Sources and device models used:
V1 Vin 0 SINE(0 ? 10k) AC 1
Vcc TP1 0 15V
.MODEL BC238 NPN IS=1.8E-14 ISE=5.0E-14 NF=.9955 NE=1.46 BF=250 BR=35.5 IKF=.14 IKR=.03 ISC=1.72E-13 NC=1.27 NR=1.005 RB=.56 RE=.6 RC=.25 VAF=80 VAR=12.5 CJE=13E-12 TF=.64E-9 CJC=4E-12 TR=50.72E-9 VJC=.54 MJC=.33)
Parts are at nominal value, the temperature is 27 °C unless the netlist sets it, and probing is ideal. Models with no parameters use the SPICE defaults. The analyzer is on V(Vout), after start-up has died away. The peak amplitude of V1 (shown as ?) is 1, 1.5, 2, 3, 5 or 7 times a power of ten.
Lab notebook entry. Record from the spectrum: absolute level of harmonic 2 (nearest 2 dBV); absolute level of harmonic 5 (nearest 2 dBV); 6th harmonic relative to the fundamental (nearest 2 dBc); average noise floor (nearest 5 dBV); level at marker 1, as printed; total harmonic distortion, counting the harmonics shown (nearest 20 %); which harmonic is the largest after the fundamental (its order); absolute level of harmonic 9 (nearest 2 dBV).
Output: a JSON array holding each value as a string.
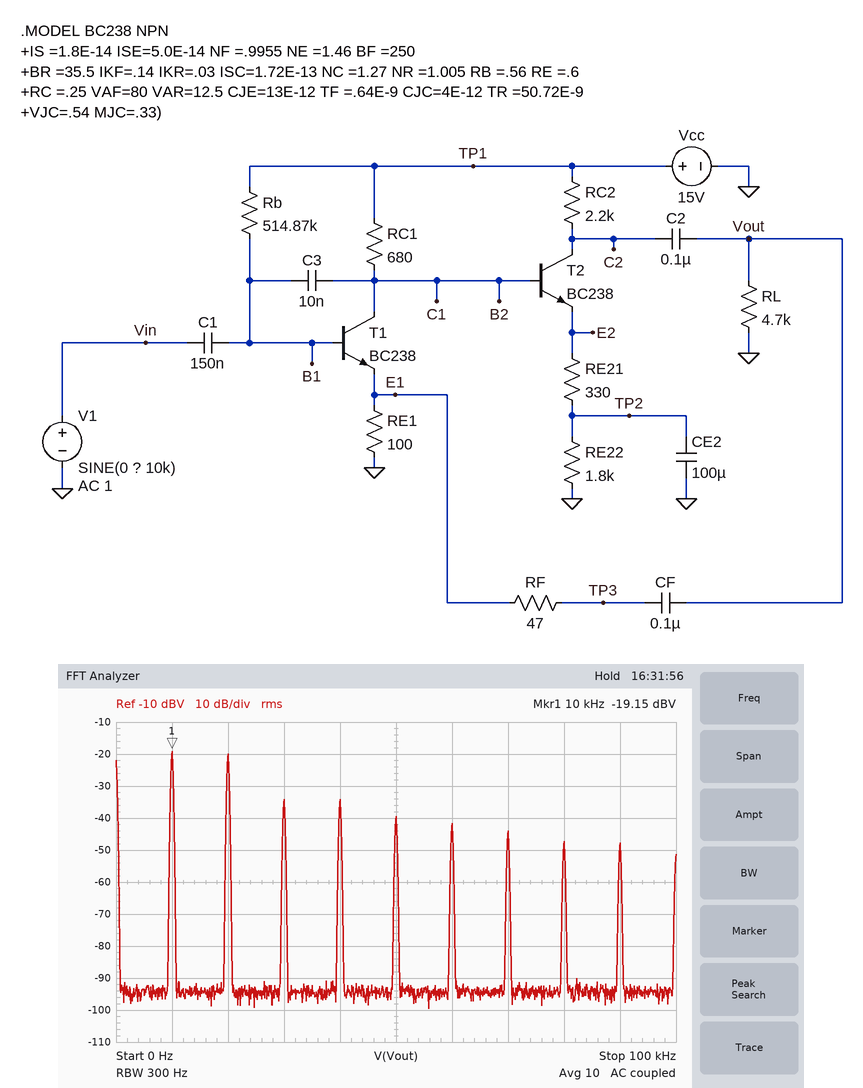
["-20 dBV", "-40 dBV", "-22 dBc", "-95 dBV", "-19.15 dBV", "100 %", "2", "-48 dBV"]
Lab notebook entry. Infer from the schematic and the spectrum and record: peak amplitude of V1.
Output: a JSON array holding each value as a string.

["500 mV"]
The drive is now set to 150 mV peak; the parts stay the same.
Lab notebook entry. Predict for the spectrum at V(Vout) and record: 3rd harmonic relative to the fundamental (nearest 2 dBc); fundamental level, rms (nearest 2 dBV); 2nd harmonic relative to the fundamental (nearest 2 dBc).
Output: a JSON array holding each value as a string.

["-34 dBc", "-28 dBV", "-28 dBc"]
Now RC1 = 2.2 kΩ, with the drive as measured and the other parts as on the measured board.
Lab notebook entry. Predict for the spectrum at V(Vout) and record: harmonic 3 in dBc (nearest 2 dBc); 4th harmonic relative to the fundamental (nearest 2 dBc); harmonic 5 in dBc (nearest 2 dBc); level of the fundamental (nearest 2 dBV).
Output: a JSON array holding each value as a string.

["-26 dBc", "-42 dBc", "-36 dBc", "-8 dBV"]
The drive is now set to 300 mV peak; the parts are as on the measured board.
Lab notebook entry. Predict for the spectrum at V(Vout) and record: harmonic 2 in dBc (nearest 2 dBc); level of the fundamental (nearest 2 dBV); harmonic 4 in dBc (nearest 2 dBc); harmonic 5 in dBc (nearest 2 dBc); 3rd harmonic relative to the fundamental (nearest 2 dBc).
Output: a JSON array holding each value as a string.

["4 dBc", "-32 dBV", "-12 dBc", "-12 dBc", "-4 dBc"]
